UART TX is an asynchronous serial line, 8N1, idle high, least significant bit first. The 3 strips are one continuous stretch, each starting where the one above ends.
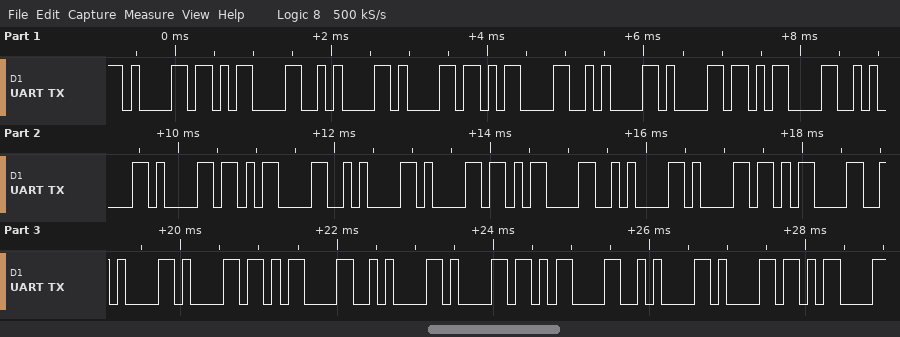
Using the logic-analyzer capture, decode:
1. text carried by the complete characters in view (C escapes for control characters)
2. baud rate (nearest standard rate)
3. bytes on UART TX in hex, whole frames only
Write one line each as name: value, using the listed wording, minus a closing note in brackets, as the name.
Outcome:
text carried by the complete characters in view: "a\r\na\r\na\r\na\r\na\r\na\r\na\r\na\r\na\r"
baud rate: 9600 baud
bytes on UART TX in hex, whole frames only: 0x61 0x0D 0x0A 0x61 0x0D 0x0A 0x61 0x0D 0x0A 0x61 0x0D 0x0A 0x61 0x0D 0x0A 0x61 0x0D 0x0A 0x61 0x0D 0x0A 0x61 0x0D 0x0A 0x61 0x0D
